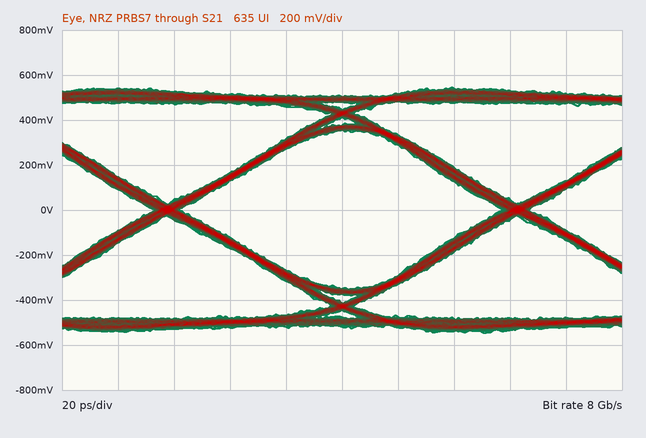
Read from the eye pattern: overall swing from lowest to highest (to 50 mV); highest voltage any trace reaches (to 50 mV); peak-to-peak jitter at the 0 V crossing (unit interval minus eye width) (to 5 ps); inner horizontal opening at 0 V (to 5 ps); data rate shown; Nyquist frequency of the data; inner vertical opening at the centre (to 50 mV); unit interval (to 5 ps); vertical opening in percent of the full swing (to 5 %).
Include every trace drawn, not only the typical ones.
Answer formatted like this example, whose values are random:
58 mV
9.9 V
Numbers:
1.10 V
550 mV
10 ps
115 ps
8 Gb/s
4 GHz
700 mV
125 ps
65 %
